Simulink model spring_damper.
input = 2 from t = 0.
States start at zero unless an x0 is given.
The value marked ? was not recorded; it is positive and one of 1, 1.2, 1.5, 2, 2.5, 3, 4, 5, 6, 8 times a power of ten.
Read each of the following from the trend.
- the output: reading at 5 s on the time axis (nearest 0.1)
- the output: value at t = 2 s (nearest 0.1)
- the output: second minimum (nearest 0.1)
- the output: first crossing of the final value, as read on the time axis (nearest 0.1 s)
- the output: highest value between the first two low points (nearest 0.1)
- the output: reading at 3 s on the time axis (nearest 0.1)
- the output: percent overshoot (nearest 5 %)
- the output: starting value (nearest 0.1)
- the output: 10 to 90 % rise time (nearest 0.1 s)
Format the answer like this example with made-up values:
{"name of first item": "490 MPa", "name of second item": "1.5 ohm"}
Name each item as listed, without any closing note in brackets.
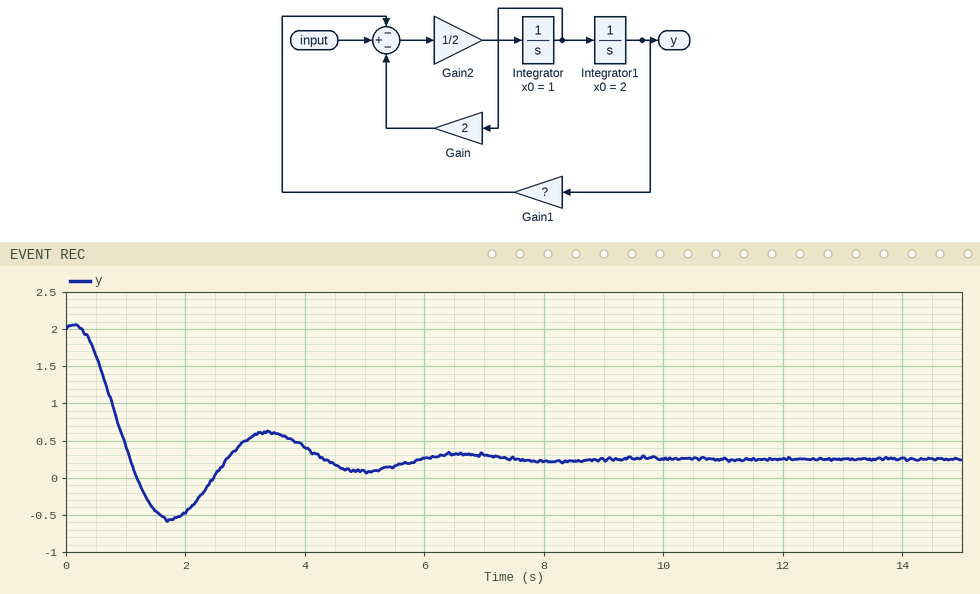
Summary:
{"the output: reading at 5 s on the time axis": "0.1", "the output: value at t = 2 s": "-0.5", "the output: second minimum": "0.1", "the output: first crossing of the final value, as read on the time axis": "1.1 s", "the output: highest value between the first two low points": "0.6", "the output: reading at 3 s on the time axis": "0.5", "the output: percent overshoot": "45 %", "the output: starting value": "2.0", "the output: 10 to 90 % rise time": "0.6 s"}
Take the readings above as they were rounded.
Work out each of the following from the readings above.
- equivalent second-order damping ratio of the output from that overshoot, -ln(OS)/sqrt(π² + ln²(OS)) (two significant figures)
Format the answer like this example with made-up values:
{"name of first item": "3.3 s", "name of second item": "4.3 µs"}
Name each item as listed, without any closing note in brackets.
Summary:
{"equivalent second-order damping ratio of the output from that overshoot, -ln(OS)/sqrt(π² + ln²(OS))": "0.25"}
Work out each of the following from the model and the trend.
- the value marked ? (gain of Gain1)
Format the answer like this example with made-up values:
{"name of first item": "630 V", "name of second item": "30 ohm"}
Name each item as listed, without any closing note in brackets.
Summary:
{"the value marked ?": "8"}
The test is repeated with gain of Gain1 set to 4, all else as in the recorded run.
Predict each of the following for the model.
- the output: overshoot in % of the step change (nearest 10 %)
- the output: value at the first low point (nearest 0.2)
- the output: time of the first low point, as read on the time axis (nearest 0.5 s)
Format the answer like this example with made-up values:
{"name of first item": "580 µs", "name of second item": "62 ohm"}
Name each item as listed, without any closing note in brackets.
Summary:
{"the output: overshoot in % of the step change": "30 %", "the output: value at the first low point": "0.0", "the output: time of the first low point, as read on the time axis": "2.5 s"}
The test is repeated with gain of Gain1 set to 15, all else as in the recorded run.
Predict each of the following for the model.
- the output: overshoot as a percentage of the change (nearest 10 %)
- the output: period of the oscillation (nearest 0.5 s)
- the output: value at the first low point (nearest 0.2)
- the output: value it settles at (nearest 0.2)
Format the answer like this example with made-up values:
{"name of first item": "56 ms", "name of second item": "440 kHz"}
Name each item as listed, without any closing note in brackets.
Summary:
{"the output: overshoot as a percentage of the change": "60 %", "the output: period of the oscillation": "2.5 s", "the output: value at the first low point": "-1.0", "the output: value it settles at": "0.2"}
